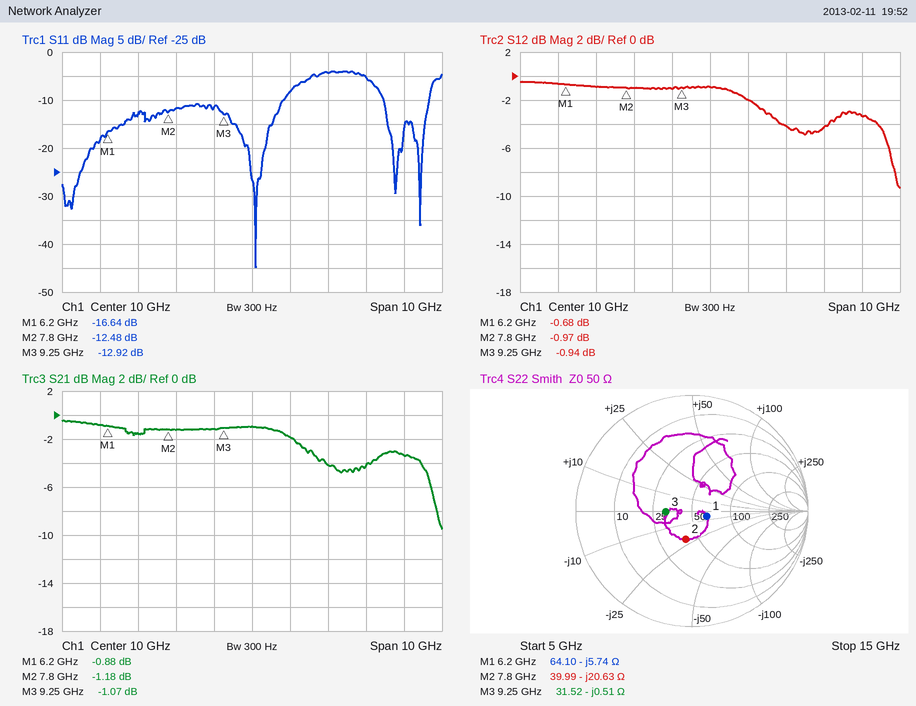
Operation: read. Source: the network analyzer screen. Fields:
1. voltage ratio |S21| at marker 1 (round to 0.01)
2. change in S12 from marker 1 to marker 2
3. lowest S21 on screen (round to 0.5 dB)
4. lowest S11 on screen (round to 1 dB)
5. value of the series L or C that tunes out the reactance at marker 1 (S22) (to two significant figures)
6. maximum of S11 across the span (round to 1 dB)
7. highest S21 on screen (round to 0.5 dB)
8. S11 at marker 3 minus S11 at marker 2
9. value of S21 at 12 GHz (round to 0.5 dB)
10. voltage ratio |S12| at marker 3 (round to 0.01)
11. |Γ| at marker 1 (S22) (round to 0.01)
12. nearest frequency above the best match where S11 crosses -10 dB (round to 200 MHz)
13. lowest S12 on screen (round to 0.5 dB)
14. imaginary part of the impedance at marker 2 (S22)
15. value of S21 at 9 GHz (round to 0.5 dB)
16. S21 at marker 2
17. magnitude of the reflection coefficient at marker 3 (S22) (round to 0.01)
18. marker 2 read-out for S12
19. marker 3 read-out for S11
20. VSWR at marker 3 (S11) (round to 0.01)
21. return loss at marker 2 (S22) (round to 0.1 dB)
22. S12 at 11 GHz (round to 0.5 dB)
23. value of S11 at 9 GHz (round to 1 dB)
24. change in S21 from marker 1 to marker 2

0.90
-0.29 dB
-9.5 dB
-45 dB
150 pH
-4 dB
-0.5 dB
-0.44 dB
-4.0 dB
0.90
0.13
10.8 GHz
-9.5 dB
-20.63 Ω
-1.0 dB
-1.18 dB
0.23
-0.97 dB
-12.92 dB
1.58
12.1 dB
-2.0 dB
-12 dB
-0.30 dB
